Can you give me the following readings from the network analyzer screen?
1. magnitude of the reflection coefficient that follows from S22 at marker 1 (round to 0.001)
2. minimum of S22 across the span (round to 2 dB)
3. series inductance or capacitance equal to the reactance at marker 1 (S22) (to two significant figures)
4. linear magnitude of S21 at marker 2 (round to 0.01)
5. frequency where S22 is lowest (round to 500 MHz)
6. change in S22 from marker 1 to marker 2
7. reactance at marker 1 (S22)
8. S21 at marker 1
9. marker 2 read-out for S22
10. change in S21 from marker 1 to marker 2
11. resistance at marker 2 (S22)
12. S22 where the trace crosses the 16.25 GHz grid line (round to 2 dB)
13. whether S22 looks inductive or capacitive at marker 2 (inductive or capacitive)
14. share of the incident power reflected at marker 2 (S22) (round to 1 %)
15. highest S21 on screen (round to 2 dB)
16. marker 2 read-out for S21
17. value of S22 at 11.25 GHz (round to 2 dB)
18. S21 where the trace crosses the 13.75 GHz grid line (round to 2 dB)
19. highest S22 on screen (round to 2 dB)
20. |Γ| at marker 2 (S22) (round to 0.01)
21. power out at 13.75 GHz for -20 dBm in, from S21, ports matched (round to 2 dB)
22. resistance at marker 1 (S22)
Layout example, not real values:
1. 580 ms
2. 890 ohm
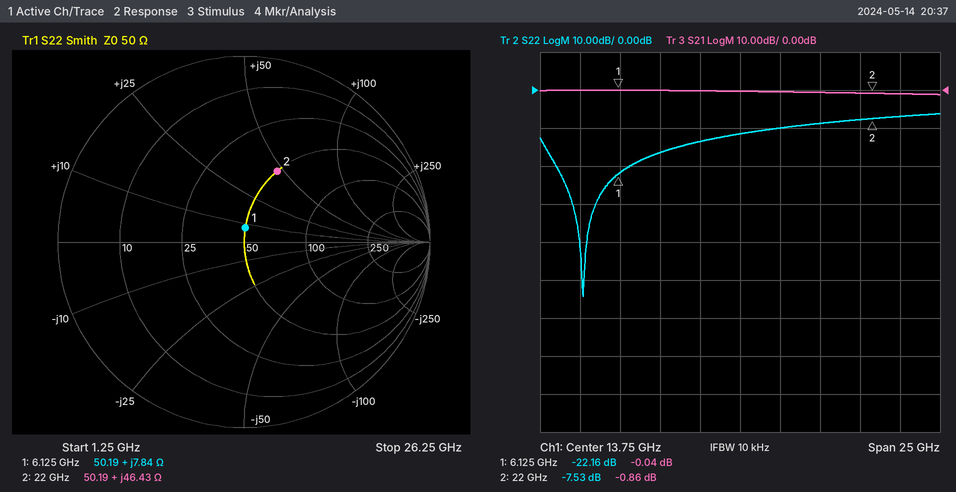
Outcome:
1. 0.078
2. -54 dB
3. 200 pH
4. 0.91
5. 4.0 GHz
6. 14.63 dB
7. +7.84 Ω
8. -0.04 dB
9. -7.53 dB
10. -0.82 dB
11. 50.19 Ω
12. -10 dB
13. inductive
14. 18 %
15. 0 dB
16. -0.86 dB
17. -14 dB
18. 0 dB
19. -6 dB
20. 0.42
21. -20 dBm
22. 50.19 Ω
